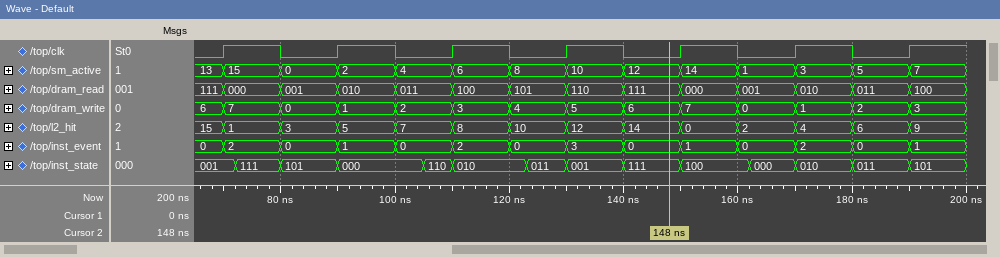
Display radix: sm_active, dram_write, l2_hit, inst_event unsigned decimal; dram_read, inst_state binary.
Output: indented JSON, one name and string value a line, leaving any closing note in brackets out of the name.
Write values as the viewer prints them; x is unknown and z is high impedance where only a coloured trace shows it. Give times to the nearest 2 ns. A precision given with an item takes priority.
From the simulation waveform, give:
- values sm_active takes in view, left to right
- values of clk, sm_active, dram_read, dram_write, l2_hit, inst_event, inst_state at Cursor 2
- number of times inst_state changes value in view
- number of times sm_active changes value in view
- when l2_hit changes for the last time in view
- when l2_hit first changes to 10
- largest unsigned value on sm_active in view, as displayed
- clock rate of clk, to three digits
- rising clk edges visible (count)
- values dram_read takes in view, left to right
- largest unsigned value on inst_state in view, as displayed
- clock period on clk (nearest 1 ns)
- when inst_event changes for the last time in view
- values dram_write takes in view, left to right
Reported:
{
  "values sm_active takes in view, left to right": "13, 15, 0, 2, 4, 6, 8, 10, 12, 14, 1, 3, 5, 7",
  "values of clk, sm_active, dram_read, dram_write, l2_hit, inst_event, inst_state at Cursor 2": "clk=0, sm_active=12, dram_read=111, dram_write=6, l2_hit=14, inst_event=0, inst_state=111",
  "number of times inst_state changes value in view": "13",
  "number of times sm_active changes value in view": "13",
  "when l2_hit changes for the last time in view": "190 ns",
  "when l2_hit first changes to 10": "120 ns",
  "largest unsigned value on sm_active in view, as displayed": "15",
  "clock rate of clk, to three digits": "50.0 MHz",
  "rising clk edges visible": "7",
  "values dram_read takes in view, left to right": "111, 000, 001, 010, 011, 100, 101, 110, 111, 000, 001, 010, 011, 100",
  "largest unsigned value on inst_state in view, as displayed": "111",
  "clock period on clk": "20 ns",
  "when inst_event changes for the last time in view": "190 ns",
  "values dram_write takes in view, left to right": "6, 7, 0, 1, 2, 3, 4, 5, 6, 7, 0, 1, 2, 3"
}
